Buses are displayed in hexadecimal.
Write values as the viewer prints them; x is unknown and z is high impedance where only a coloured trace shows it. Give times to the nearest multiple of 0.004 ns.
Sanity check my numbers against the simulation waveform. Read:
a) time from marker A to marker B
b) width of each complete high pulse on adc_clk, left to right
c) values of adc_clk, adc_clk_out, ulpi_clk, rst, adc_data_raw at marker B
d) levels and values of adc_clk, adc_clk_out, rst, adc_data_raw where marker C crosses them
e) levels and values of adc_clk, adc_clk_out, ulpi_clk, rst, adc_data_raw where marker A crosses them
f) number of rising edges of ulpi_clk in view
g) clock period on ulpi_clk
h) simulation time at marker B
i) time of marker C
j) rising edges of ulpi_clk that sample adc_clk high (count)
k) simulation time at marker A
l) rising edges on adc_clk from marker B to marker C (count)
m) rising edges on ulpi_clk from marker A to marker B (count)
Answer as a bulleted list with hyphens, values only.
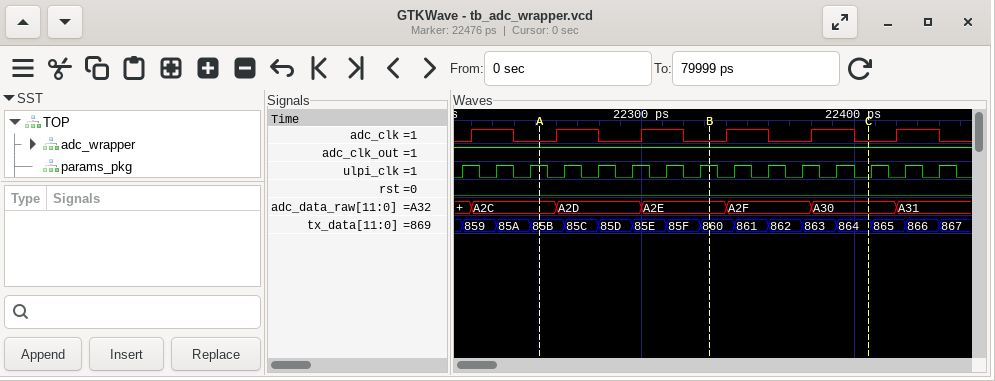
- 0.08 ns
- 0.02 ns, 0.02 ns, 0.02 ns, 0.02 ns, 0.02 ns, 0.02 ns
- adc_clk=0, adc_clk_out=1, ulpi_clk=1, rst=0, adc_data_raw=A2E
- adc_clk=0, adc_clk_out=1, rst=0, adc_data_raw=A30
- adc_clk=0, adc_clk_out=1, ulpi_clk=1, rst=0, adc_data_raw=A2C
- 15
- 0.016 ns
- 22.332 ns
- 22.408 ns
- 9
- 22.252 ns
- 2
- 5
